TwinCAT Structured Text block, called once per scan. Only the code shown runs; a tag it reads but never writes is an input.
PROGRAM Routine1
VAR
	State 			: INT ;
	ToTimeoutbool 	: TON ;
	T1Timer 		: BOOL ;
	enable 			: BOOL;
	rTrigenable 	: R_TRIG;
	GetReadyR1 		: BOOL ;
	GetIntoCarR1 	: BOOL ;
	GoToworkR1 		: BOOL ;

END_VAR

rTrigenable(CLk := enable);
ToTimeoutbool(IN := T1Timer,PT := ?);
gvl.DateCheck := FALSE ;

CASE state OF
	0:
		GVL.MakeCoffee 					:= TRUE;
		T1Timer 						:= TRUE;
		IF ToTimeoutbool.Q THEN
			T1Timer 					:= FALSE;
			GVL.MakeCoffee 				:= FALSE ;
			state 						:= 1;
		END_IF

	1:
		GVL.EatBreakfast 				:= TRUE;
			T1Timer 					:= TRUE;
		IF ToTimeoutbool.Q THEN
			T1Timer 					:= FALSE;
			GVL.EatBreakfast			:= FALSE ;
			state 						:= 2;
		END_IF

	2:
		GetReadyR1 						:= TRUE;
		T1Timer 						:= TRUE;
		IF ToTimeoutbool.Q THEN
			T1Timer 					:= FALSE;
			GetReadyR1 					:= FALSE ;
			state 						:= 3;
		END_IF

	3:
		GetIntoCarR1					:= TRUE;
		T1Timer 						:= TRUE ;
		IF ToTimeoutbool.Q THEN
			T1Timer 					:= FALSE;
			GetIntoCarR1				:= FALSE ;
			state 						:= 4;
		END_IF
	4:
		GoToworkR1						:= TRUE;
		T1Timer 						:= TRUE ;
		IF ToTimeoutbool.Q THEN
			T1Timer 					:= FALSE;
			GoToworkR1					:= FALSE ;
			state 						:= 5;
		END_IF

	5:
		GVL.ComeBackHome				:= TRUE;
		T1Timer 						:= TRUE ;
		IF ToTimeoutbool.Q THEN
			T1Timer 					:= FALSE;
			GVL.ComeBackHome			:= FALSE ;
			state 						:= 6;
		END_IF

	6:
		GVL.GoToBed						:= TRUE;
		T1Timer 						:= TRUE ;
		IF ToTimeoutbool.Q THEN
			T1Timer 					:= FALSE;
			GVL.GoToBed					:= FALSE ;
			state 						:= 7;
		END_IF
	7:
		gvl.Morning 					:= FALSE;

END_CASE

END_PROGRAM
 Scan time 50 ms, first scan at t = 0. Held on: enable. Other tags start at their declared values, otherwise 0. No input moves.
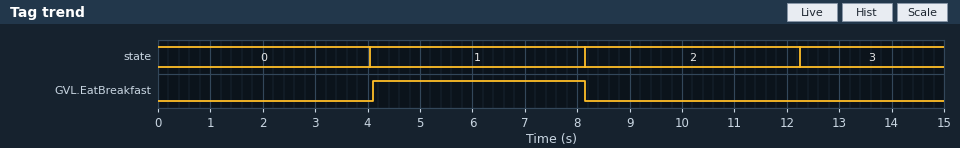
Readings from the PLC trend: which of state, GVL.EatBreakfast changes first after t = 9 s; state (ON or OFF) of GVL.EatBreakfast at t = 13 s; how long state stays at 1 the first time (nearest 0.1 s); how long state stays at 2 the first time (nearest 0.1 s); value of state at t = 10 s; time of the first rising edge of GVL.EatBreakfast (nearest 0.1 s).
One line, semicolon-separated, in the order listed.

state; OFF; 4.1 s; 4.1 s; 2; 4.1 s
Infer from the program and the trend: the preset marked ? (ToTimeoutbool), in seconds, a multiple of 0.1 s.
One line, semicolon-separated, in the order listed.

4.0 s
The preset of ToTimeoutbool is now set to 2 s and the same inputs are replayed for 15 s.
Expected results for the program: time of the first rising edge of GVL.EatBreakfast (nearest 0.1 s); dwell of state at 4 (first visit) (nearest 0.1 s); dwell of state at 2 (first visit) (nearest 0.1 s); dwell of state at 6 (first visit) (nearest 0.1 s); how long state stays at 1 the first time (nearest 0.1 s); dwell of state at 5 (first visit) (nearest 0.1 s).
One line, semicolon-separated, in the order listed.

2.1 s; 2.1 s; 2.1 s; 2.1 s; 2.1 s; 2.1 s
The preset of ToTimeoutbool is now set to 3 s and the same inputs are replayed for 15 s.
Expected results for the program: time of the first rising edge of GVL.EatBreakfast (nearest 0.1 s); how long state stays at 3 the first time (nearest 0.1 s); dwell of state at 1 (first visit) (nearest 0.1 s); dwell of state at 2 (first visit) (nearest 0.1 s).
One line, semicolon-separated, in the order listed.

3.1 s; 3.1 s; 3.1 s; 3.1 s
